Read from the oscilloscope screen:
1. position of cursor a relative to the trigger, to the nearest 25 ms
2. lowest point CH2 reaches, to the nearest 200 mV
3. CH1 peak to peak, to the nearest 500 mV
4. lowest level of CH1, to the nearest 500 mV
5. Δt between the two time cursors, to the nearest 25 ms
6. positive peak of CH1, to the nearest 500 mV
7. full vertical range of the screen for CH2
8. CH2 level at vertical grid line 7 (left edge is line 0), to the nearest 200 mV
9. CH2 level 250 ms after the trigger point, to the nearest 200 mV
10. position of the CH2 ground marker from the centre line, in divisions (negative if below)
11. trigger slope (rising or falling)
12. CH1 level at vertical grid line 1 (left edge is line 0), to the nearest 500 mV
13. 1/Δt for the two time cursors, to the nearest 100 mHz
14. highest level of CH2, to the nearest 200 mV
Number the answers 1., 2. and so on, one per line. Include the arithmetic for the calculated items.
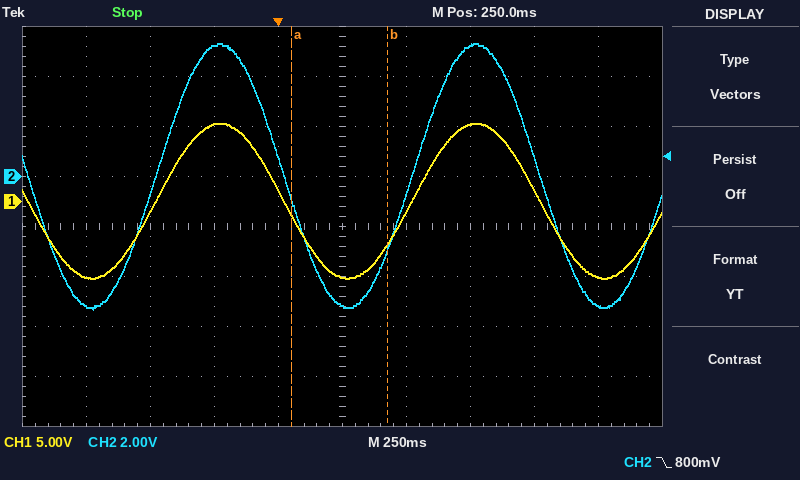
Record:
1. +50 ms
2. -5.4 V
3. 8.0 V − (-7.5 V) = 15.5 V
4. -7.5 V
5. 375 ms
6. 8.0 V
7. 16 V
8. 5.2 V
9. -5.2 V
10. +1.0 div
11. falling
12. -7.5 V
13. 1 / 375 ms ≈ 2.7 Hz
14. 5.4 V
